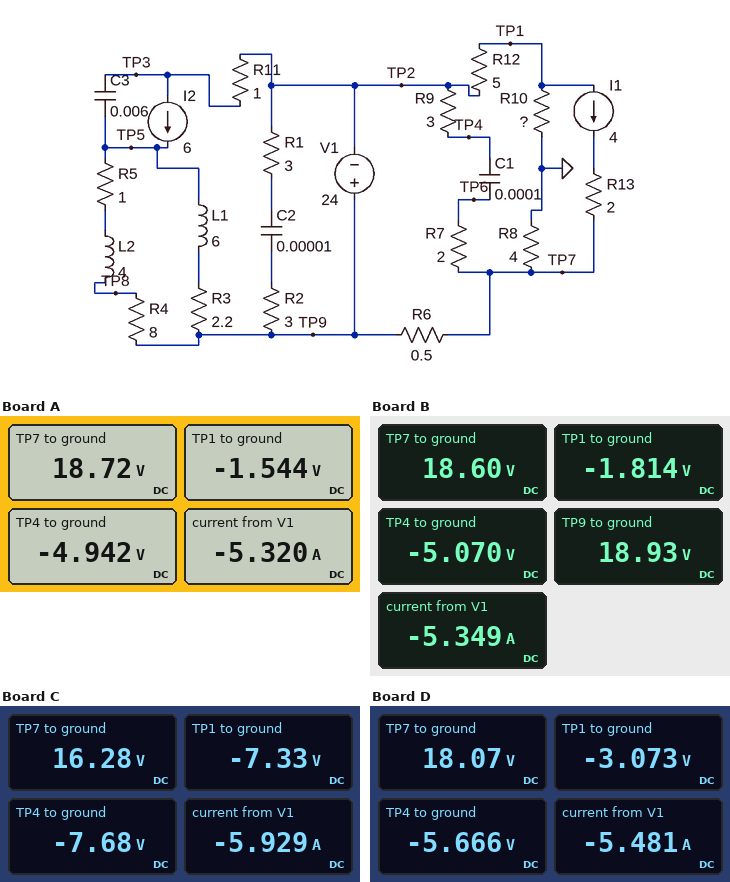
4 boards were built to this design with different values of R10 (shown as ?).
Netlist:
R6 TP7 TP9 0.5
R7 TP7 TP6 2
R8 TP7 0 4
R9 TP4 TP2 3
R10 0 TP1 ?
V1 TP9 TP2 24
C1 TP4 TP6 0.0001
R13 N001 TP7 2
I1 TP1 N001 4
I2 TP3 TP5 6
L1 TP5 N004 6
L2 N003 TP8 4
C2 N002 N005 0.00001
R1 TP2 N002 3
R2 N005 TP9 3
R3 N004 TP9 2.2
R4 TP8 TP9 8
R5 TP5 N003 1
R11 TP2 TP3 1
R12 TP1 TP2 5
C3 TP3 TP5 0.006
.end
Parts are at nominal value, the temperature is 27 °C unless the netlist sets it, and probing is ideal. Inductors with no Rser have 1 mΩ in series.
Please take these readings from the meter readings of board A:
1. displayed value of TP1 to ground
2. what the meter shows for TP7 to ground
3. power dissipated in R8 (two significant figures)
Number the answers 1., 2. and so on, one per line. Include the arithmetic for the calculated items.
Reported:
1. -1.544 V
2. 18.72 V
3. (18.72 V)^2 / 4 Ω = 88 W
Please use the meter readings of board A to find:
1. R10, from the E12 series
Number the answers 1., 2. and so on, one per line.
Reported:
1. 0.33 Ω
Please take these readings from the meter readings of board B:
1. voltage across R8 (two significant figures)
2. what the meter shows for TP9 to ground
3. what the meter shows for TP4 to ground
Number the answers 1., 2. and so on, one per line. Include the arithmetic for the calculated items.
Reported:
1. 18.6 V = 19 V
2. 18.93 V
3. -5.070 V
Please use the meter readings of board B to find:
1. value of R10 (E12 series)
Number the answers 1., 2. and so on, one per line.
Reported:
1. 0.39 Ω
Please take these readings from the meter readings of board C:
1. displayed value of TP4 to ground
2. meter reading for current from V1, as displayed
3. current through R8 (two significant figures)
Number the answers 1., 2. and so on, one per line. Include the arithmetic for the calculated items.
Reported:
1. -7.68 V
2. -5.929 A
3. (16.28 V) / 4 Ω = 4.1 A
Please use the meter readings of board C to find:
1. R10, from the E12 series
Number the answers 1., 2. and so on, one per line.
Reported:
1. 1.8 Ω
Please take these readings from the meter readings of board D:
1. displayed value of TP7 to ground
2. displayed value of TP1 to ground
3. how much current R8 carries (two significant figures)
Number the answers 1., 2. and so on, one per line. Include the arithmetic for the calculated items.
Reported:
1. 18.07 V
2. -3.073 V
3. (18.07 V) / 4 Ω = 4.5 A
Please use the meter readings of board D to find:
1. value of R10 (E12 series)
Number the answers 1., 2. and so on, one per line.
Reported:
1. 0.68 Ω
